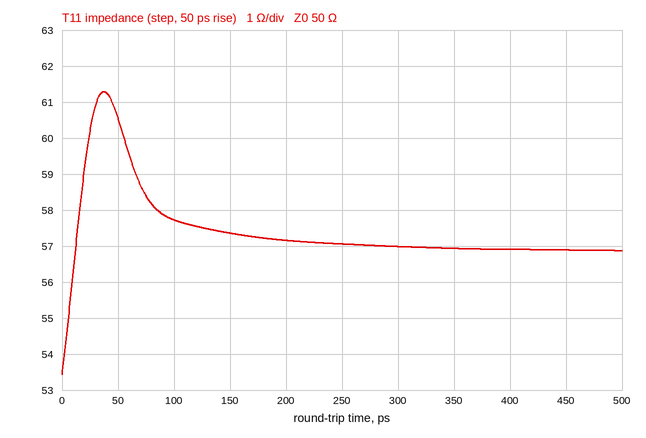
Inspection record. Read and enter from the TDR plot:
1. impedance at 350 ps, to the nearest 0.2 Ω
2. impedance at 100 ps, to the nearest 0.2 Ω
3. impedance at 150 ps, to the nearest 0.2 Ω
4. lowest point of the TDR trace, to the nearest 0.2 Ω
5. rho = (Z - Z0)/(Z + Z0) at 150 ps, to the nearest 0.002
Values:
57.0 Ω
57.8 Ω
57.4 Ω
53.4 Ω
+0.068
